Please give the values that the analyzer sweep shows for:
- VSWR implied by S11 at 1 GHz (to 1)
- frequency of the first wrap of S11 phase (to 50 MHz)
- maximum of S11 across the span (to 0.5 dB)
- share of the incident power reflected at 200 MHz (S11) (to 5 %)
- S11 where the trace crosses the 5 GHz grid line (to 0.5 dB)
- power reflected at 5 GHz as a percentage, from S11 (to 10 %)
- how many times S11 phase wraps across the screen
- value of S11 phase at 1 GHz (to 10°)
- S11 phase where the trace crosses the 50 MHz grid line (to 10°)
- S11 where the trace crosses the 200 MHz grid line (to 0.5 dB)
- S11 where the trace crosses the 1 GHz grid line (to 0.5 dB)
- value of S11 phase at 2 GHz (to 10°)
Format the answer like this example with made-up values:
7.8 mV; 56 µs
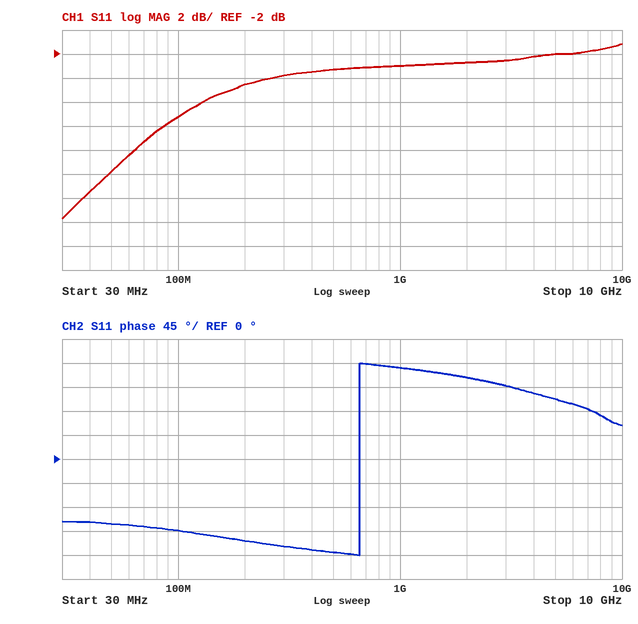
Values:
6; 650 MHz; -1.0 dB; 35 %; -2.0 dB; 60 %; 1; 170°; -120°; -4.5 dB; -3.0 dB; 150°
